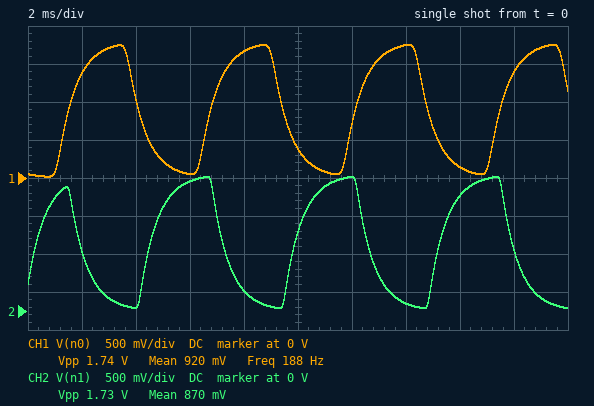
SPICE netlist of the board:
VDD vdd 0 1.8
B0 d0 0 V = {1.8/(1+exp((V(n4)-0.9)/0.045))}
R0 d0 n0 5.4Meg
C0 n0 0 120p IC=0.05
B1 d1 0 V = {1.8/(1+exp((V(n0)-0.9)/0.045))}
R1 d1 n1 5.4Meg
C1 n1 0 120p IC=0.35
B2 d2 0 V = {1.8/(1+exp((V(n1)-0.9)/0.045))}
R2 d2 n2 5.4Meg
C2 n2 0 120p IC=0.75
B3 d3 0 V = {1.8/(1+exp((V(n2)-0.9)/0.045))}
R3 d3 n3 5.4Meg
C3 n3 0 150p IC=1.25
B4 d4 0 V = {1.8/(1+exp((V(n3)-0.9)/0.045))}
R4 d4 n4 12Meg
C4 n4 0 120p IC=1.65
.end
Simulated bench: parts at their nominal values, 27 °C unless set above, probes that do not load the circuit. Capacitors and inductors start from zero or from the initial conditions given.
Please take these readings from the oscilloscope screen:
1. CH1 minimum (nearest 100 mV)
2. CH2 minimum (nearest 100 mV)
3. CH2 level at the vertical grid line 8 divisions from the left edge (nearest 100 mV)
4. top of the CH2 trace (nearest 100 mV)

0 V
0 V
1.5 V
1.8 V
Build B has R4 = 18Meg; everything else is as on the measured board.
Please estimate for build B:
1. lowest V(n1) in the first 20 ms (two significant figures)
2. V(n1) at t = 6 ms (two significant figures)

25 mV
1.5 V
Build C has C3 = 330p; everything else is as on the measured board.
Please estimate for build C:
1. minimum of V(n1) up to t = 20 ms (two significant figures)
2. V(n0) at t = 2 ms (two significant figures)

17 mV
1.5 V
